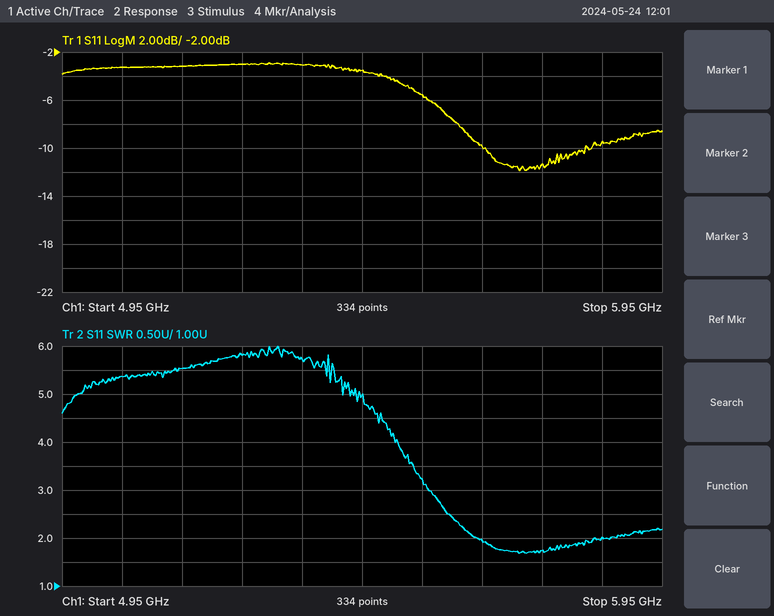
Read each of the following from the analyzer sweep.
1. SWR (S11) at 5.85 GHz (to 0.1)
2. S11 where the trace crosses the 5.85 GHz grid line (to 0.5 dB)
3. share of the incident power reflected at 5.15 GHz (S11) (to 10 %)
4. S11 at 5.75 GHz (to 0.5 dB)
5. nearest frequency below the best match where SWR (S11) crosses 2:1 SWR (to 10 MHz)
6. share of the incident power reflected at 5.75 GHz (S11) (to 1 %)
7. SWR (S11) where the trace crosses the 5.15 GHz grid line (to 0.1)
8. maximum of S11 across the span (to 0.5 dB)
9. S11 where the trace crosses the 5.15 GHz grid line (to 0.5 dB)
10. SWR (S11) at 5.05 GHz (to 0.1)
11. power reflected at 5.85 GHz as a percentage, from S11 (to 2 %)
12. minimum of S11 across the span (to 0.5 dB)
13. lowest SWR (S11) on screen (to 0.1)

2.0
-9.5 dB
50 %
-11.5 dB
5.64 GHz
7 %
5.5
-3.0 dB
-3.0 dB
5.4
12 %
-12.0 dB
1.7
